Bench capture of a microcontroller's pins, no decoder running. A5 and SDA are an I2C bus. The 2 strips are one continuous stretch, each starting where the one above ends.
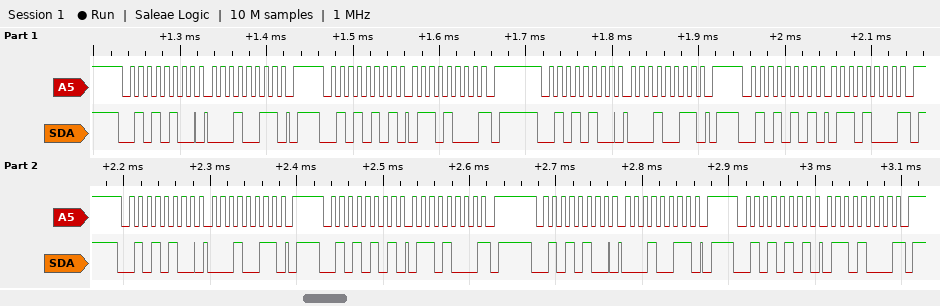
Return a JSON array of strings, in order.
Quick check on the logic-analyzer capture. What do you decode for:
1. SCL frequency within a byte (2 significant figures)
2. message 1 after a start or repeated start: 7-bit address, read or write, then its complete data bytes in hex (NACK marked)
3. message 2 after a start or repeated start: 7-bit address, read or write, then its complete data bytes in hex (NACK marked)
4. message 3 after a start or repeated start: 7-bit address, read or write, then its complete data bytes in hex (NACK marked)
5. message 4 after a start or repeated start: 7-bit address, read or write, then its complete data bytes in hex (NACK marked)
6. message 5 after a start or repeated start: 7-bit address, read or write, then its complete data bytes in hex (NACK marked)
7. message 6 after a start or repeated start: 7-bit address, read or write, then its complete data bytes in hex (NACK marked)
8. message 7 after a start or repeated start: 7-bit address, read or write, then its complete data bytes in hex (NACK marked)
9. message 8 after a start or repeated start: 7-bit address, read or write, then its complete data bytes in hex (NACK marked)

["100 kHz", "0x2A write: 13", "0x2A read: 68 NACK", "0x2A write: 13", "0x2A read: 68 NACK", "0x2A write: 13", "0x2A read: 68 NACK", "0x2A write: 13", "0x2A read: 68 NACK"]
